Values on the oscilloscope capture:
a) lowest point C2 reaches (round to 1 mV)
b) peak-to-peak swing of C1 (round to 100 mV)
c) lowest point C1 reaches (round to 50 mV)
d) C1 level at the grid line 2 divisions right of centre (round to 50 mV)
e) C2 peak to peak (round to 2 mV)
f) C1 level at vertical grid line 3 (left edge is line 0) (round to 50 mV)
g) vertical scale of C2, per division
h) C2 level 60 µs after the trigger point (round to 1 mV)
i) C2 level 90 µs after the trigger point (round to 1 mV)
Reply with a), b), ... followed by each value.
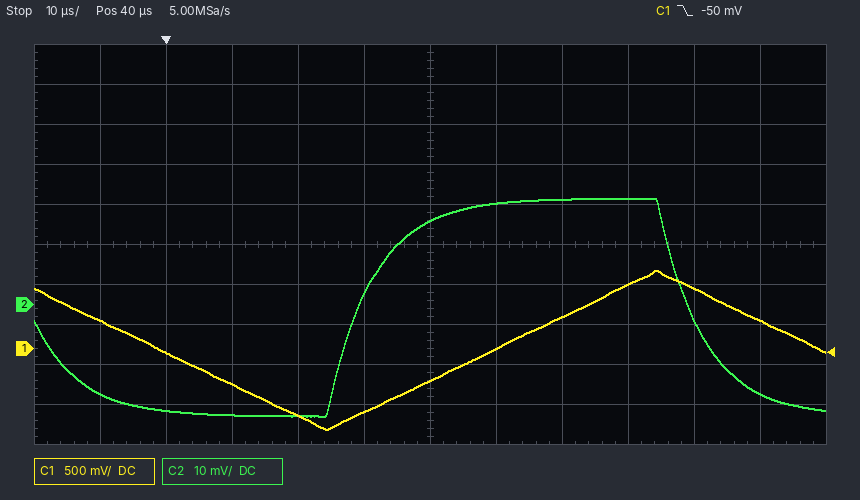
a) -28 mV
b) 2.00 V
c) -1.00 V
d) 400 mV
e) 54 mV
f) -450 mV
g) 10 mV
h) 26 mV
i) -22 mV
